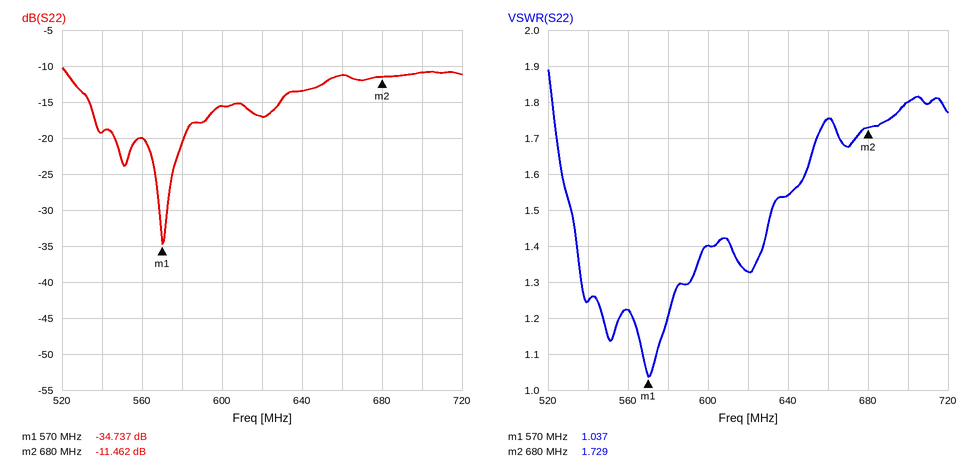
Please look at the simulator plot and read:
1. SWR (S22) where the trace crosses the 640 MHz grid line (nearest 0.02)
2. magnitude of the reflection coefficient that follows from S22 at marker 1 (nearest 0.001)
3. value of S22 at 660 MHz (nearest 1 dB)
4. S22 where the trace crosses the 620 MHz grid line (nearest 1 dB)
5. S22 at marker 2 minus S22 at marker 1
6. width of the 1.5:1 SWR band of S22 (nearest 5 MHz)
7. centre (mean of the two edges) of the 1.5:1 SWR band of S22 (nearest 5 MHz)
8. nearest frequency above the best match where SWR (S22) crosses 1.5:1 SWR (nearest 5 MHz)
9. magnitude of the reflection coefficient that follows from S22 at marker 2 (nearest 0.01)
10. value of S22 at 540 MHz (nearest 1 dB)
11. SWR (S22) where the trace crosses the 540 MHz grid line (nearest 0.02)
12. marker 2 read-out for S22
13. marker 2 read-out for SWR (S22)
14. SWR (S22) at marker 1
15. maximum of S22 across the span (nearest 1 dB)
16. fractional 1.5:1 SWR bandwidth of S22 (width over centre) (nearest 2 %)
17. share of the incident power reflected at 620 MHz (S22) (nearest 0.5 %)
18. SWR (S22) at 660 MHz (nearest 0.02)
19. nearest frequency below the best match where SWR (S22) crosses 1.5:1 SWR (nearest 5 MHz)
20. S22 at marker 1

1.54
0.018
-11 dB
-17 dB
23.275 dB
100 MHz
580 MHz
630 MHz
0.27
-19 dB
1.24
-11.462 dB
1.729
1.037
-10 dB
18 %
2.0 %
1.76
530 MHz
-34.737 dB
